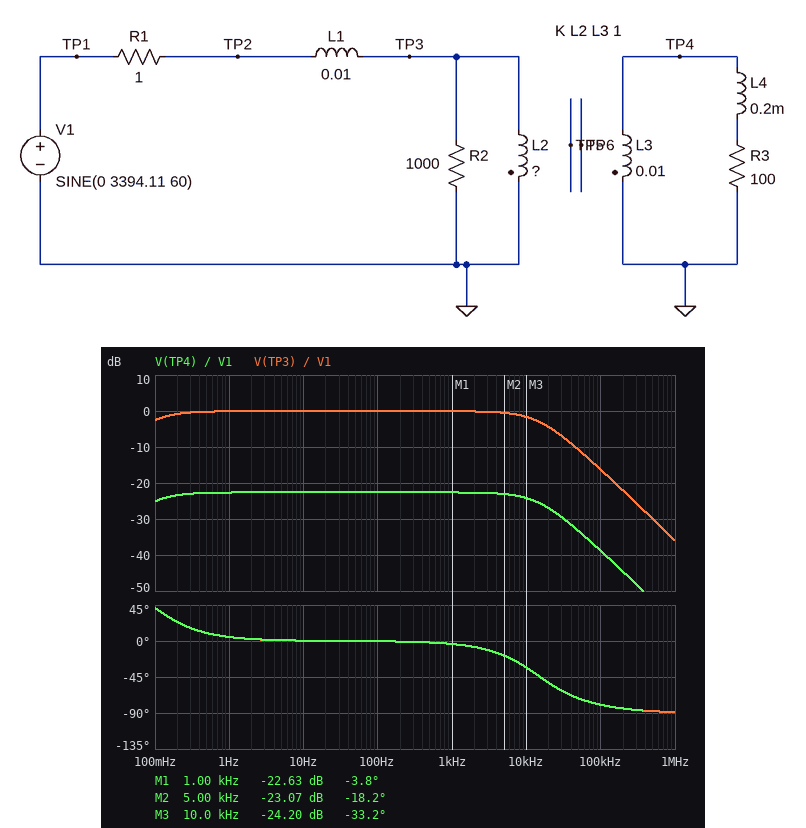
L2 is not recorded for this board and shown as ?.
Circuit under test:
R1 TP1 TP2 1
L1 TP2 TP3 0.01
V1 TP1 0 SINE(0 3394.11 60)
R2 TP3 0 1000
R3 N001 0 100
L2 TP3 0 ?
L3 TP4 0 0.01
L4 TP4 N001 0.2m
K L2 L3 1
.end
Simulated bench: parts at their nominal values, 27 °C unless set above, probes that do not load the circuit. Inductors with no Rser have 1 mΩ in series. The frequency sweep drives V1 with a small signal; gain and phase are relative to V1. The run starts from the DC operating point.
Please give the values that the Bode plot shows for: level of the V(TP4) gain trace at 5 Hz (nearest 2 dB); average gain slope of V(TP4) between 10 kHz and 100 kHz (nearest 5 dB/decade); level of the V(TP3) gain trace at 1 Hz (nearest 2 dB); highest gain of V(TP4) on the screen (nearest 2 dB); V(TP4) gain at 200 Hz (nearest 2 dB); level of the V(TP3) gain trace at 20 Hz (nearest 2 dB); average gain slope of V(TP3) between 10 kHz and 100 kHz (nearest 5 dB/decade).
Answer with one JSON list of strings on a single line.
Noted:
["-22 dB", "-15 dB/decade", "0 dB", "-22 dB", "-22 dB", "0 dB", "-15 dB/decade"]
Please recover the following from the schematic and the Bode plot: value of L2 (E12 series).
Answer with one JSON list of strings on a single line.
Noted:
["1.8 H"]
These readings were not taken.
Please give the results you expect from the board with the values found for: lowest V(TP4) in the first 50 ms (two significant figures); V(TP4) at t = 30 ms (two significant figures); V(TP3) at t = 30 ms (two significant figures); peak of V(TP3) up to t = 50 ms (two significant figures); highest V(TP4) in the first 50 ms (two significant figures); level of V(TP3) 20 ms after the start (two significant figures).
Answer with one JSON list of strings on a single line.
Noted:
["-250 V", "-240 V", "-3.2 kV", "3.4 kV", "250 V", "3.2 kV"]
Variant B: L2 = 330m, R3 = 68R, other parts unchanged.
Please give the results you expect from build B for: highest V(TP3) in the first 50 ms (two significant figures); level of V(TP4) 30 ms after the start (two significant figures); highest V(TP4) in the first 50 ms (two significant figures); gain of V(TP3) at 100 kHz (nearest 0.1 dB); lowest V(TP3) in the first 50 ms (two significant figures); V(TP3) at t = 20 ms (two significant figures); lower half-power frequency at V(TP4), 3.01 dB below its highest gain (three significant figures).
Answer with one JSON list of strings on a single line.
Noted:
["3.3 kV", "-550 V", "570 V", "-17.2 dB", "-3.3 kV", "3.1 kV", "468 mHz"]
